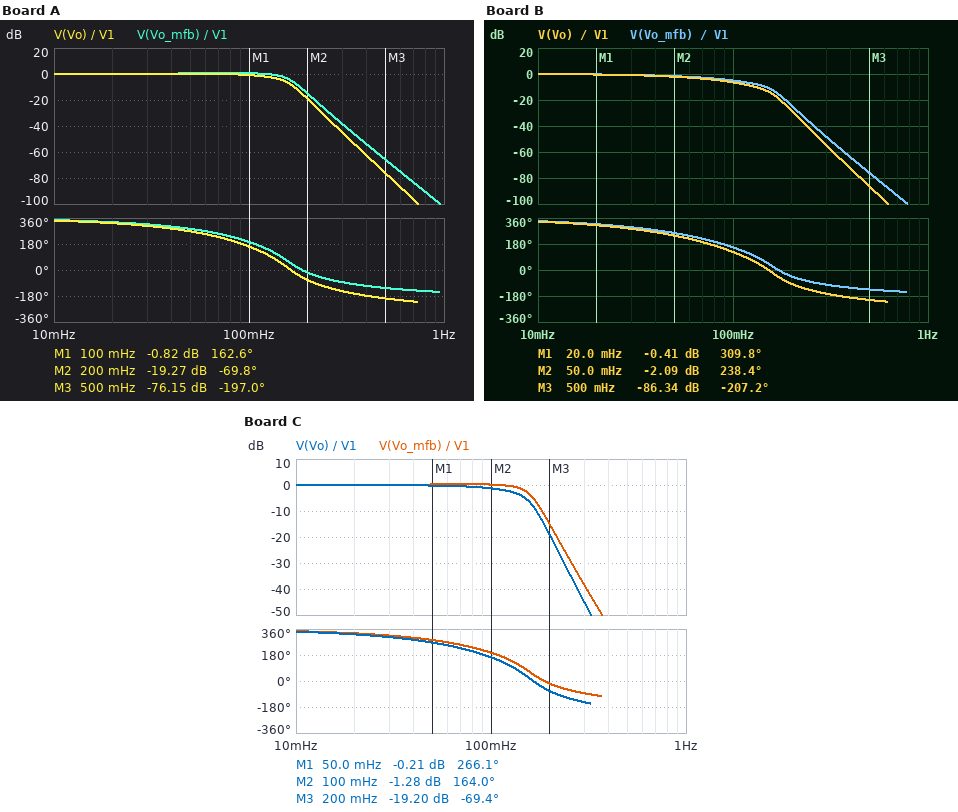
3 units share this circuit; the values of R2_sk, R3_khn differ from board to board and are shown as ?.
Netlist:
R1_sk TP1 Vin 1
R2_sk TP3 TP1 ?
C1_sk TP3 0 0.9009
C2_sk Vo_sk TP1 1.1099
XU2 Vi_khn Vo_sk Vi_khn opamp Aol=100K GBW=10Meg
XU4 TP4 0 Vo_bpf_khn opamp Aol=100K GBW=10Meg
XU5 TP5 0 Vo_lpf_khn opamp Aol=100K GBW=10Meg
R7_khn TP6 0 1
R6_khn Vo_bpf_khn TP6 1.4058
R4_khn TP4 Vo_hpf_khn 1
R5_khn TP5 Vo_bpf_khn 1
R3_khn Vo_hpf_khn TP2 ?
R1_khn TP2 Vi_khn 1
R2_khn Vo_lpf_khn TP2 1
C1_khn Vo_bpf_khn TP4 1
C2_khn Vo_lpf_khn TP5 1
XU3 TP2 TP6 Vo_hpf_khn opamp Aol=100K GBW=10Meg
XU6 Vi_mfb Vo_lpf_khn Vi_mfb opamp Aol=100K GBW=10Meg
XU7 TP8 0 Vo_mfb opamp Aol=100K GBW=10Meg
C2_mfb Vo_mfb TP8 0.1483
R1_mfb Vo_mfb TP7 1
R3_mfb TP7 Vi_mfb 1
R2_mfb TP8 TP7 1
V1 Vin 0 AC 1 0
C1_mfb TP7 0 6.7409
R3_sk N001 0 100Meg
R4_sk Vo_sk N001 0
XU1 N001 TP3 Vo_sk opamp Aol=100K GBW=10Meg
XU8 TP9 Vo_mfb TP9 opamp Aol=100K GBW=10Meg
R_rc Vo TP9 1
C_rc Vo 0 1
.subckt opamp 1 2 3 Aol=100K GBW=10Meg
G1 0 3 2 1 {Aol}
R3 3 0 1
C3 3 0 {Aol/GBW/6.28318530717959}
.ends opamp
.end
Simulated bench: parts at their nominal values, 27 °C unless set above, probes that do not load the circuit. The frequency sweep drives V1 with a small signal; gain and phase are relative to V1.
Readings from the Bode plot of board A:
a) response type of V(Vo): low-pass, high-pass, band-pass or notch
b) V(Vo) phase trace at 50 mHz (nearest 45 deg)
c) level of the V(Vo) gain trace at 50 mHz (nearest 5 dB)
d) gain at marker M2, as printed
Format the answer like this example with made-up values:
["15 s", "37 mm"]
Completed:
["low-pass", "270 deg", "0 dB", "-19.27 dB"]
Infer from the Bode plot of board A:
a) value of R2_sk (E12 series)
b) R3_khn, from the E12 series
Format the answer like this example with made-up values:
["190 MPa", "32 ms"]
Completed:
["1.2 Ω", "0.56 Ω"]
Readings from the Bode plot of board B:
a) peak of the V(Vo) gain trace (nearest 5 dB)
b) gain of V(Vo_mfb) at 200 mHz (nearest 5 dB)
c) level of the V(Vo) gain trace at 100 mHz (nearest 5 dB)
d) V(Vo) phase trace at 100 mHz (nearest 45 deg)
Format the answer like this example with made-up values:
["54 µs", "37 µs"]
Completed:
["0 dB", "-25 dB", "-5 dB", "135 deg"]
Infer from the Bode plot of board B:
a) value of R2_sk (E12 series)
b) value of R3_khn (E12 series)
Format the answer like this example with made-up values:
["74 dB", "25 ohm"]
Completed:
["3.3 Ω", "0.47 Ω"]
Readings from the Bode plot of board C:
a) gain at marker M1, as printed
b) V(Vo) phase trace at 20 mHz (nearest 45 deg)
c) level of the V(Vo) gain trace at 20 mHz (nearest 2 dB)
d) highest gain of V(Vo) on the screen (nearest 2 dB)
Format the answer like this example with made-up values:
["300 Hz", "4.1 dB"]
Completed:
["-0.21 dB", "315 deg", "0 dB", "0 dB"]
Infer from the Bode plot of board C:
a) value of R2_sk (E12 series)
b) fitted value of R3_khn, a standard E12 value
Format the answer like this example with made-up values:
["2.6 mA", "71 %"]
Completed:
["1.5 Ω", "0.68 Ω"]
